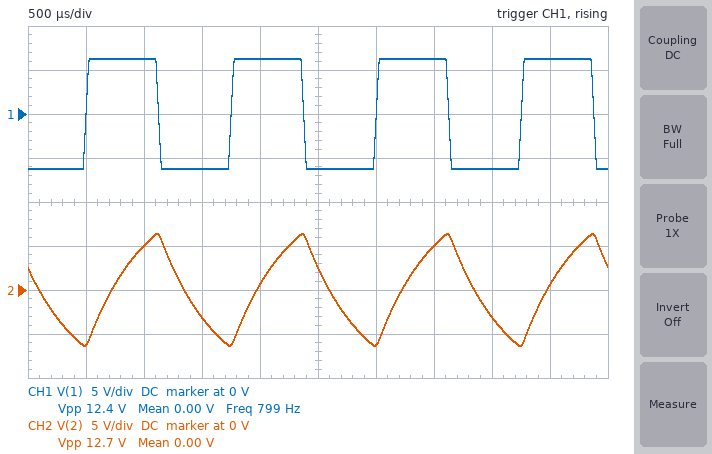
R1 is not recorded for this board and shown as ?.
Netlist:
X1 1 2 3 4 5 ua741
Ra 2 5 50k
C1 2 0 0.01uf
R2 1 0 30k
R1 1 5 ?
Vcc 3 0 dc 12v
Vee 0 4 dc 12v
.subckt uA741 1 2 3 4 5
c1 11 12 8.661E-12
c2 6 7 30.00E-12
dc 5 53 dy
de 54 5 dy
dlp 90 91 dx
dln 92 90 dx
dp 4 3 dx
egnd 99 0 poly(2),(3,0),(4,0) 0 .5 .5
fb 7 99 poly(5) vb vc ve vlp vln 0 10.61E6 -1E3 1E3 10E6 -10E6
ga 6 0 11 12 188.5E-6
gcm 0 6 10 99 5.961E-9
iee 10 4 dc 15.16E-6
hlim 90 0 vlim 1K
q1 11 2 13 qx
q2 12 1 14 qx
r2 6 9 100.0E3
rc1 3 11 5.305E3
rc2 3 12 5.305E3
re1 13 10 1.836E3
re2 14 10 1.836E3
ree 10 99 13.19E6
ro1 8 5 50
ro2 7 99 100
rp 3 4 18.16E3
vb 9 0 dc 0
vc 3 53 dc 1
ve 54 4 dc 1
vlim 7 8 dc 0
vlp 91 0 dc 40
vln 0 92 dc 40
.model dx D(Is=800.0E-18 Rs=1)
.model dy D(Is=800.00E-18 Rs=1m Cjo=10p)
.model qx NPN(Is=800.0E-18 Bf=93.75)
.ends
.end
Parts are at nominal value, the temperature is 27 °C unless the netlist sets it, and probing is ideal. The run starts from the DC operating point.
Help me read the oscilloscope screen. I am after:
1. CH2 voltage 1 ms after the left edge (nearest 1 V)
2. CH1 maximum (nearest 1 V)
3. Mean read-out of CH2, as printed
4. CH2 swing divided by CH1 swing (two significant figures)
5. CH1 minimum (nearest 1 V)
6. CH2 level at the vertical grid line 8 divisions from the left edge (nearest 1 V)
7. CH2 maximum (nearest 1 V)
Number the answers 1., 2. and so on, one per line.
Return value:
1. 5 V
2. 6 V
3. 0.00 V
4. 1.0
5. -6 V
6. -3 V
7. 6 V
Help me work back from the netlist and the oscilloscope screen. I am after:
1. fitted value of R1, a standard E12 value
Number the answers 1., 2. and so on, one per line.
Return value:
1. 27 kΩ
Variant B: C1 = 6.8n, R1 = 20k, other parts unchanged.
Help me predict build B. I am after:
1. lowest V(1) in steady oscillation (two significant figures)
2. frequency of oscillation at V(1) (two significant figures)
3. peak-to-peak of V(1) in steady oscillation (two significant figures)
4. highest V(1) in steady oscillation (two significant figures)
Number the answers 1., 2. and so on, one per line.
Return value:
1. -7.1 V
2. 980 Hz
3. 14 V
4. 7.1 V
